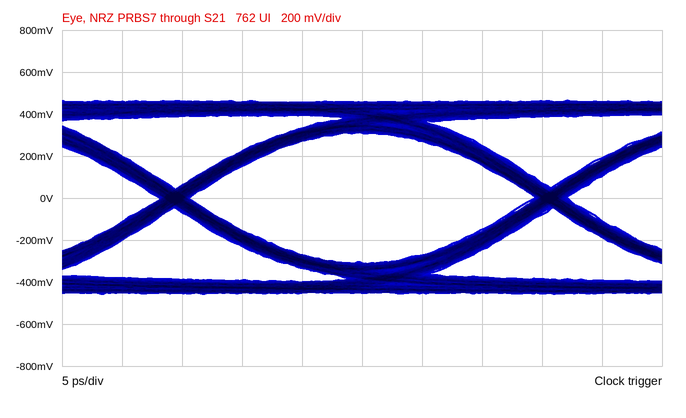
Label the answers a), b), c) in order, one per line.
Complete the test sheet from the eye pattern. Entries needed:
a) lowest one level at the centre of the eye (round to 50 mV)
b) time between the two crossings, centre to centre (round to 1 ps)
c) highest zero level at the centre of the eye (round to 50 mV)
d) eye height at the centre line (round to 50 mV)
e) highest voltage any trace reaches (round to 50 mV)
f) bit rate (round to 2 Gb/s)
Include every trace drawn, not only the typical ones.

a) 300 mV
b) 31 ps
c) -300 mV
d) 600 mV
e) 450 mV
f) 32 Gb/s
